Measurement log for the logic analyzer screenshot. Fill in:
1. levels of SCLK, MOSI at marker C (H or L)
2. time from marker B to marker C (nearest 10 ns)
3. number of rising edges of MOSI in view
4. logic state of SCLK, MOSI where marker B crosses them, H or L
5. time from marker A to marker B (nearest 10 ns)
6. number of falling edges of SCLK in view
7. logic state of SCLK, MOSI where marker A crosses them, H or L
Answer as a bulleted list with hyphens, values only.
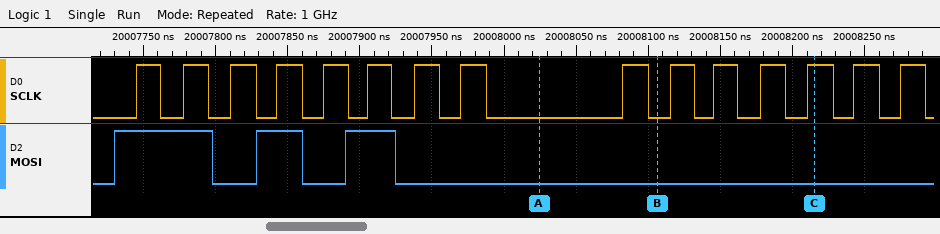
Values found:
- SCLK=H, MOSI=L
- 110 ns
- 3
- SCLK=L, MOSI=L
- 80 ns
- 15
- SCLK=L, MOSI=L
